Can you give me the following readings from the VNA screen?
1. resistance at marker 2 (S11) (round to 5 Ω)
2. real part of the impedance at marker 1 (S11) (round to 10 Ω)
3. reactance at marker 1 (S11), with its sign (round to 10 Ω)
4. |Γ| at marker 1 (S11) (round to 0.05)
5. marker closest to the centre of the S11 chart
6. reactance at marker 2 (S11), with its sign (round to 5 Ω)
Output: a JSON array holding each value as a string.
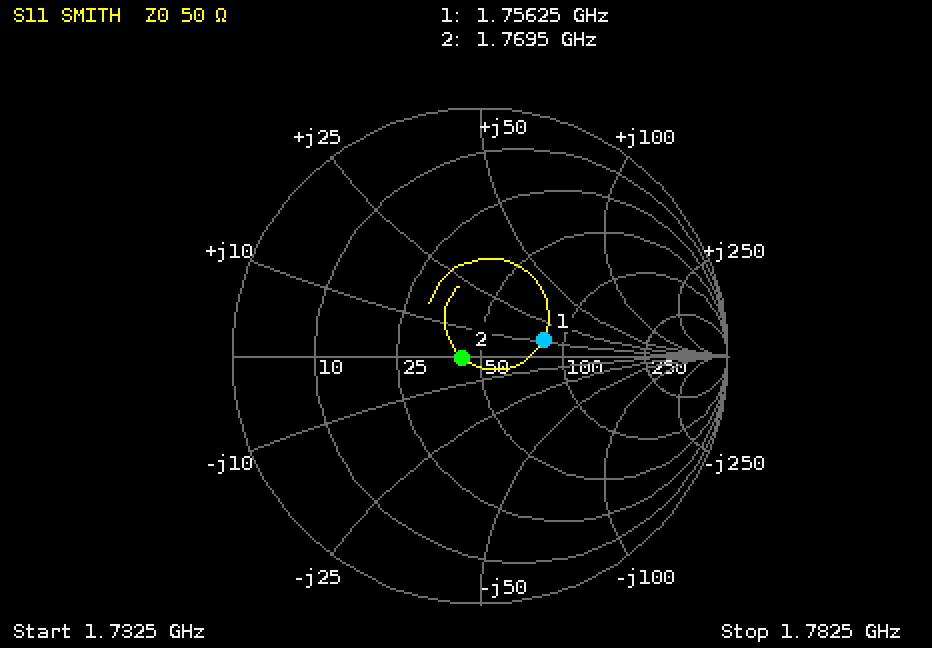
["45 Ω", "80 Ω", "+10 Ω", "0.25", "marker 2", "0 Ω"]
